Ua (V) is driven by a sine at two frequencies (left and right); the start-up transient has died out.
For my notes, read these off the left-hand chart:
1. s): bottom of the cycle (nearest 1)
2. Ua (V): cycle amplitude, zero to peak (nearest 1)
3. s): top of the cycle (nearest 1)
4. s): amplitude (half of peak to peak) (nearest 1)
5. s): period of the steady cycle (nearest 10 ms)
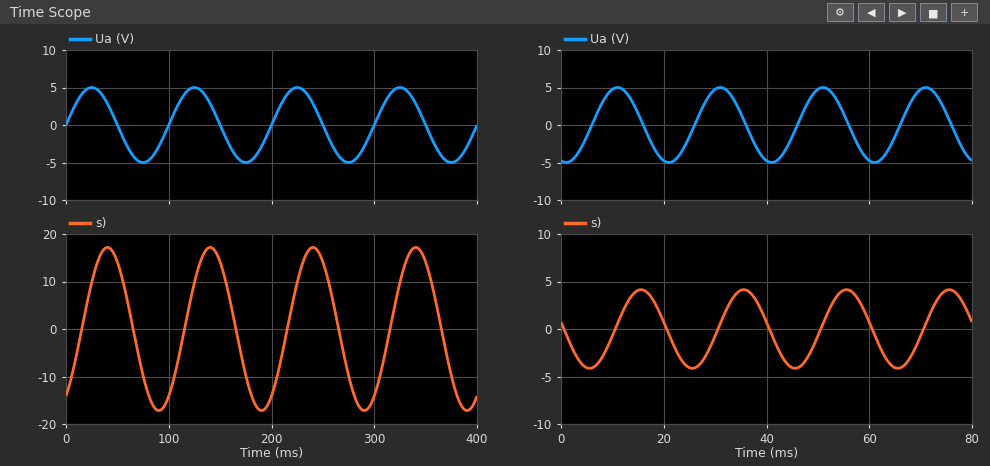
-17
5
17
17
100 ms
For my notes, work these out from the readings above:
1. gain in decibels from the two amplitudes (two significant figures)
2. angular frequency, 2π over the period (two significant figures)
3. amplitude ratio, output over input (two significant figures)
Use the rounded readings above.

11 dB
0.063 rad/ms
3.4
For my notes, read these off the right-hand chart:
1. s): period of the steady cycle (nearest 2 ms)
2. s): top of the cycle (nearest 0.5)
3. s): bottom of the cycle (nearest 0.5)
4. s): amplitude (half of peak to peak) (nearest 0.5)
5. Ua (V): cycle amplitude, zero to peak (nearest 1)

20 ms
4.0
-4.0
4.0
5
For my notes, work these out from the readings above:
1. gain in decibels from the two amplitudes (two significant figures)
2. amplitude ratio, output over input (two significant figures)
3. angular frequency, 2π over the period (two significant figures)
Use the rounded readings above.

-1.9 dB
0.80
0.31 rad/ms
